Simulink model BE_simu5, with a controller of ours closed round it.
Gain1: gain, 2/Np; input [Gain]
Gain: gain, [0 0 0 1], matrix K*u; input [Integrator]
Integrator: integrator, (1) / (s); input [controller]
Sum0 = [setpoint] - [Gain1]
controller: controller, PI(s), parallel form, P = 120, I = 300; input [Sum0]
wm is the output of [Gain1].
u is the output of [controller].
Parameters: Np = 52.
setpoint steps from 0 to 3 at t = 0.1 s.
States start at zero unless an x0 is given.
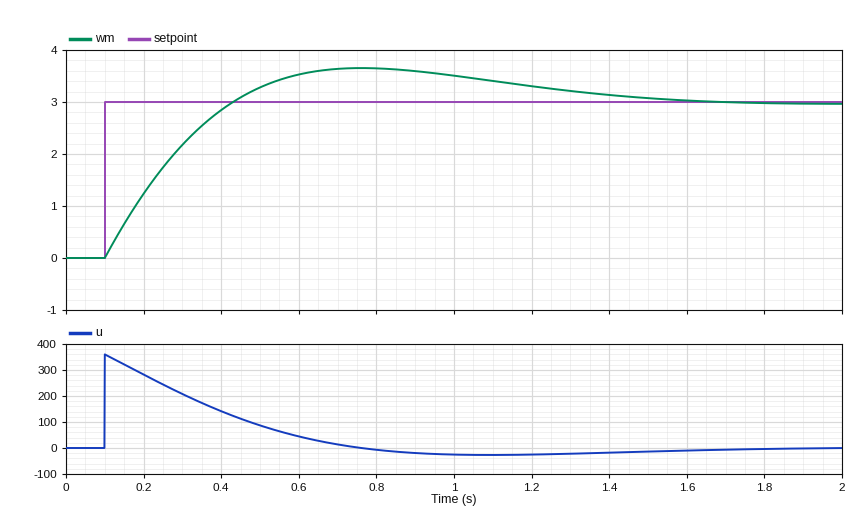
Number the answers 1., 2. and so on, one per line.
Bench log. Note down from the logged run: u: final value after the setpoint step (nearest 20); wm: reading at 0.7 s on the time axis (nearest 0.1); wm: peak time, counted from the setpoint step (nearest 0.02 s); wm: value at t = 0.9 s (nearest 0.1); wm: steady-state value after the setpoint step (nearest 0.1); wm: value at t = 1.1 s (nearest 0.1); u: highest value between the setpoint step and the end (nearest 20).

1. 0
2. 3.6
3. 0.66 s
4. 3.6
5. 3.0
6. 3.4
7. 360
